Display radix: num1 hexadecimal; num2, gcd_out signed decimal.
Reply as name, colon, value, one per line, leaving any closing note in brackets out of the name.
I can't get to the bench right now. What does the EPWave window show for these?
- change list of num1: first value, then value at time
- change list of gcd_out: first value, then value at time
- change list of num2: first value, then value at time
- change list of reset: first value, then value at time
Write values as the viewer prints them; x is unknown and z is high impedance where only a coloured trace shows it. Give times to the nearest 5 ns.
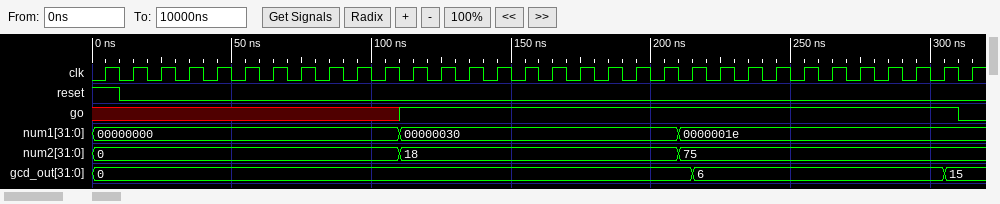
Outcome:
change list of num1: first value, then value at time: 00000000, 00000030 at 110 ns, 0000001e at 210 ns
change list of gcd_out: first value, then value at time: 0, 6 at 215 ns, 15 at 305 ns
change list of num2: first value, then value at time: 0, 18 at 110 ns, 75 at 210 ns
change list of reset: first value, then value at time: 1, 0 at 10 ns
